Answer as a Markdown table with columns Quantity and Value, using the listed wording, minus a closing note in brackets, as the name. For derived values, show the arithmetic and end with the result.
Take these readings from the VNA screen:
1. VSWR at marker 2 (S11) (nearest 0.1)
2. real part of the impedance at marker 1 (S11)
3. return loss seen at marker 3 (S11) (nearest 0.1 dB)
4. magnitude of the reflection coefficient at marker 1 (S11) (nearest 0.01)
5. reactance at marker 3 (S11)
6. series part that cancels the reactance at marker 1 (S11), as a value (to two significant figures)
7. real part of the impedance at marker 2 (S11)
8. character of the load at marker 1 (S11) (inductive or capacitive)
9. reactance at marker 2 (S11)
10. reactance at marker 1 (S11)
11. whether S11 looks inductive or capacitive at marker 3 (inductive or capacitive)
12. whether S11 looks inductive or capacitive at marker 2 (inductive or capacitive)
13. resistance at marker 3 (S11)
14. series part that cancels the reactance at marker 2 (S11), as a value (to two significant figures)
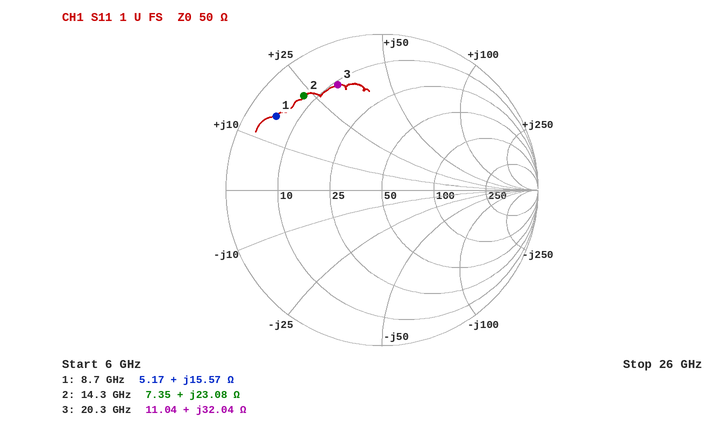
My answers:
| Quantity | Value |
|---|---|
| VSWR at marker 2 (S11) | 8.3 |
| real part of the impedance at marker 1 | 5.17 Ω |
| return loss seen at marker 3 (S11) | 2.7 dB |
| magnitude of the reflection coefficient at marker 1 (S11) | 0.83 |
| reactance at marker 3 | +32.04 Ω |
| series part that cancels the reactance at marker 1 (S11), as a value | C = 1/(2π × 8.7 GHz × 15.57 Ω) ≈ 1.2 pF |
| real part of the impedance at marker 2 | 7.35 Ω |
| character of the load at marker 1 (S11) | inductive |
| reactance at marker 2 | +23.08 Ω |
| reactance at marker 1 | +15.57 Ω |
| whether S11 looks inductive or capacitive at marker 3 | inductive |
| whether S11 looks inductive or capacitive at marker 2 | inductive |
| resistance at marker 3 | 11.04 Ω |
| series part that cancels the reactance at marker 2 (S11), as a value | C = 1/(2π × 14.3 GHz × 23.08 Ω) ≈ 482 fF, so 480 fF to two significant figures |
